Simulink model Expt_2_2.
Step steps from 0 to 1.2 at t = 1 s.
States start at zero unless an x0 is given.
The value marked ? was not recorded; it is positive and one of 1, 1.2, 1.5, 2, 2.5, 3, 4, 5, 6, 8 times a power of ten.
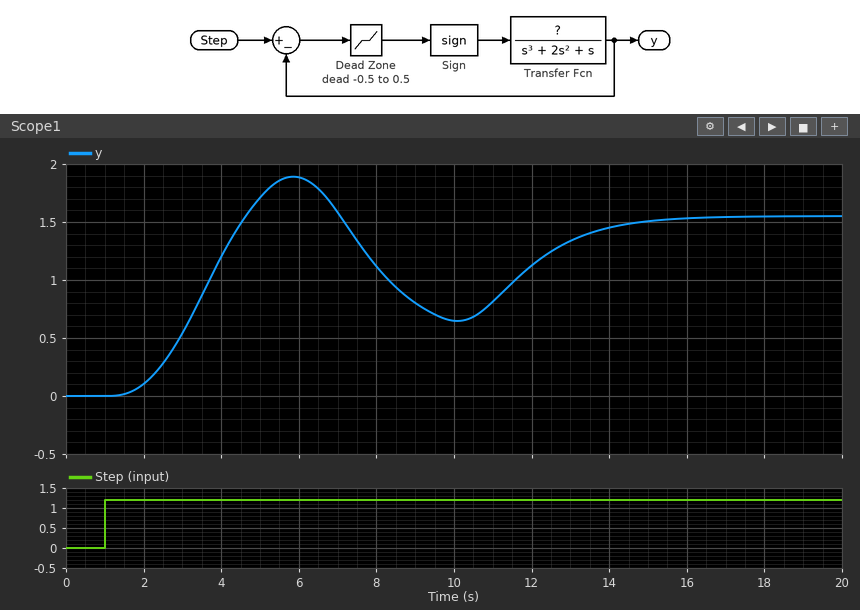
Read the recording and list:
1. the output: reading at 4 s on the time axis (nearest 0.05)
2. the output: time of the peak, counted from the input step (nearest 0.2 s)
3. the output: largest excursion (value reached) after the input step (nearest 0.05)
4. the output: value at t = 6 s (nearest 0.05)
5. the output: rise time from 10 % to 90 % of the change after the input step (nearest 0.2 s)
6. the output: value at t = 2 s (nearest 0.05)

1.20
4.8 s
1.90
1.90
2.2 s
0.10
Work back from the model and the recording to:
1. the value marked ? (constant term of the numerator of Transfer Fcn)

1
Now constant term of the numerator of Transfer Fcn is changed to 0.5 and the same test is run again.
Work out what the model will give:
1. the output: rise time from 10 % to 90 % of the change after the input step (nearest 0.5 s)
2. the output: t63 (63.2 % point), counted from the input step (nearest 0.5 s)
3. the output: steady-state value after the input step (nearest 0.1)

4.0 s
4.0 s
1.6
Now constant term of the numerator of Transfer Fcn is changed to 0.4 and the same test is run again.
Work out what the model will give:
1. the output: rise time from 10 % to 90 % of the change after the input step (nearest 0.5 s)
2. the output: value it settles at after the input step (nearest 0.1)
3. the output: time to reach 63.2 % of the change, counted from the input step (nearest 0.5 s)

4.5 s
1.4
4.0 s
